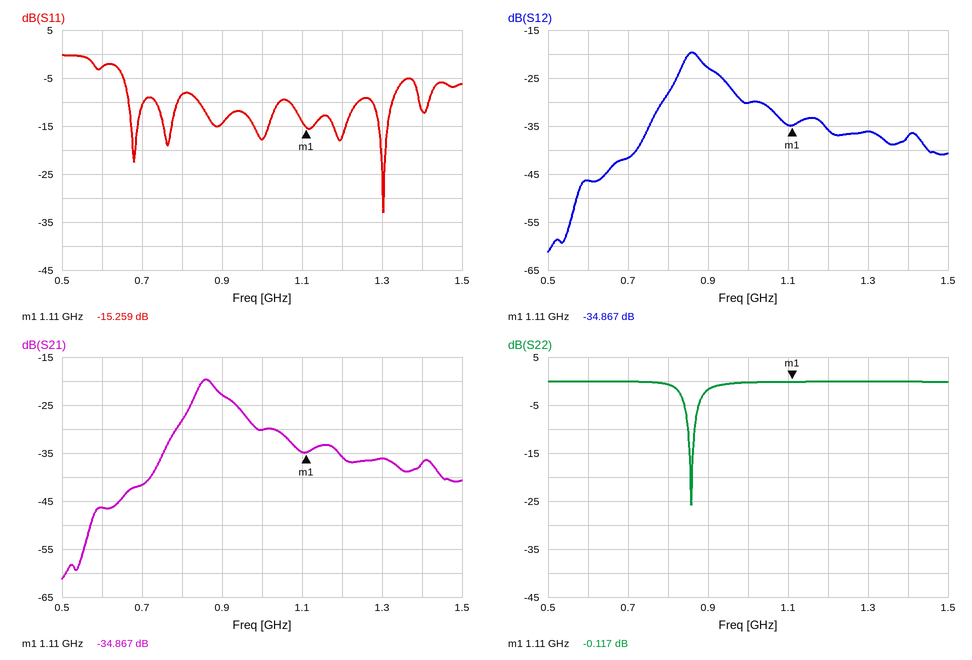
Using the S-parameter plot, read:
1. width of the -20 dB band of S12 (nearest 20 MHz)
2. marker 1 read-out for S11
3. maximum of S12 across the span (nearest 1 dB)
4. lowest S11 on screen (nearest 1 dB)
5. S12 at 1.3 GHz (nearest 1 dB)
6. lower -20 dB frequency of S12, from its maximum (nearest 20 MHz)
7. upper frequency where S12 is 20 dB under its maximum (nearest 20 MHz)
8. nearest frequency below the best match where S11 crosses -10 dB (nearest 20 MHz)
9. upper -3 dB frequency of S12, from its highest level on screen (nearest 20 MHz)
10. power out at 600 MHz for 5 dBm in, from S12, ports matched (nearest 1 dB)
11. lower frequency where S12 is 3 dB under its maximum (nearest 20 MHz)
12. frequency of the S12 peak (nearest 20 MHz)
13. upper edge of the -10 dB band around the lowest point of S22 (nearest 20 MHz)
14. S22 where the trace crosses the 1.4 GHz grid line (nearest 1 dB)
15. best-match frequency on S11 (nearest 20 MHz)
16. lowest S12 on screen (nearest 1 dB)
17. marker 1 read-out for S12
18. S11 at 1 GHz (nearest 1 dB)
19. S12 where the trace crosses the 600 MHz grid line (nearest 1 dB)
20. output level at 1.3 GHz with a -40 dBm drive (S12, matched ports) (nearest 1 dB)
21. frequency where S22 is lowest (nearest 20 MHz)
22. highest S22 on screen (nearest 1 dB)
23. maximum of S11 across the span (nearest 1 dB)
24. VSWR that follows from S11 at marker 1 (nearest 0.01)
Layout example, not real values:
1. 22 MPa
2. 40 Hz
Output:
1. 720 MHz
2. -15.259 dB
3. -20 dB
4. -33 dB
5. -36 dB
6. 720 MHz
7. 1.44 GHz
8. 1.28 GHz
9. 900 MHz
10. -41 dBm
11. 840 MHz
12. 860 MHz
13. 860 MHz
14. 0 dB
15. 1.30 GHz
16. -61 dB
17. -34.867 dB
18. -18 dB
19. -46 dB
20. -76 dBm
21. 860 MHz
22. 0 dB
23. 0 dB
24. 1.42
